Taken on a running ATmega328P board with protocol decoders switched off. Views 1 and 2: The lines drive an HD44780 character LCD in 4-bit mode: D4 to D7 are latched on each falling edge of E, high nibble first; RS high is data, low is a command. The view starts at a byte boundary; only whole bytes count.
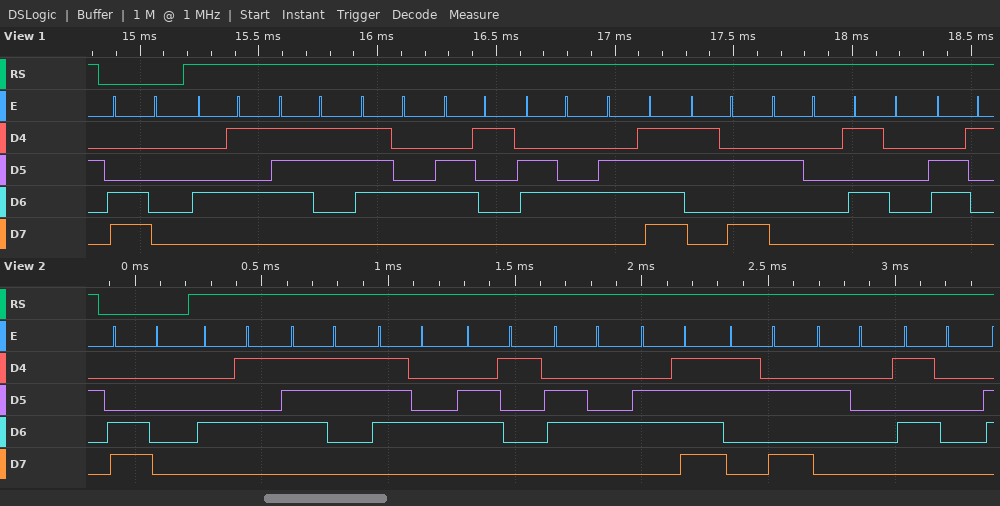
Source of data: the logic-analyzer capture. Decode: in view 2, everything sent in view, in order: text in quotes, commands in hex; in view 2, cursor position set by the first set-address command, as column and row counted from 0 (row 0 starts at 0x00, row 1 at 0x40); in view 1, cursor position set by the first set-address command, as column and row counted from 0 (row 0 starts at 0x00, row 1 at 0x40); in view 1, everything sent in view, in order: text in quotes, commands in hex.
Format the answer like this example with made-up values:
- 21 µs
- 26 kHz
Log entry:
- 0xC0 "Estado: P"
- column 0, row 1
- column 0, row 1
- 0xC0 "Estado: Pa"
